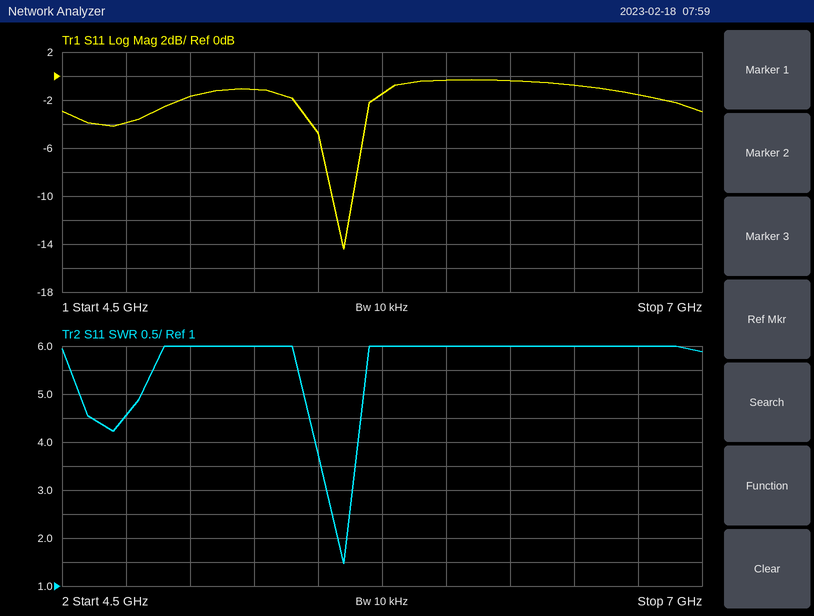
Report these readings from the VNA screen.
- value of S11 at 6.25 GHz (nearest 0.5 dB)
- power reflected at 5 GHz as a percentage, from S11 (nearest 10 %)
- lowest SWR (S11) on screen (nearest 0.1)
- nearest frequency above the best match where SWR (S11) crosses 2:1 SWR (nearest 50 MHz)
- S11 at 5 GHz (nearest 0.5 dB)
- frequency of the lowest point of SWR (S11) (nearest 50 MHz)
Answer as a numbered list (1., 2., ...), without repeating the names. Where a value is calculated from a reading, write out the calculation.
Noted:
1. -0.5 dB
2. 10^(-1.5/10) ≈ 70.8 %, so 70 % to the nearest 10 %
3. 1.5
4. 5.60 GHz
5. -1.5 dB
6. 5.60 GHz
